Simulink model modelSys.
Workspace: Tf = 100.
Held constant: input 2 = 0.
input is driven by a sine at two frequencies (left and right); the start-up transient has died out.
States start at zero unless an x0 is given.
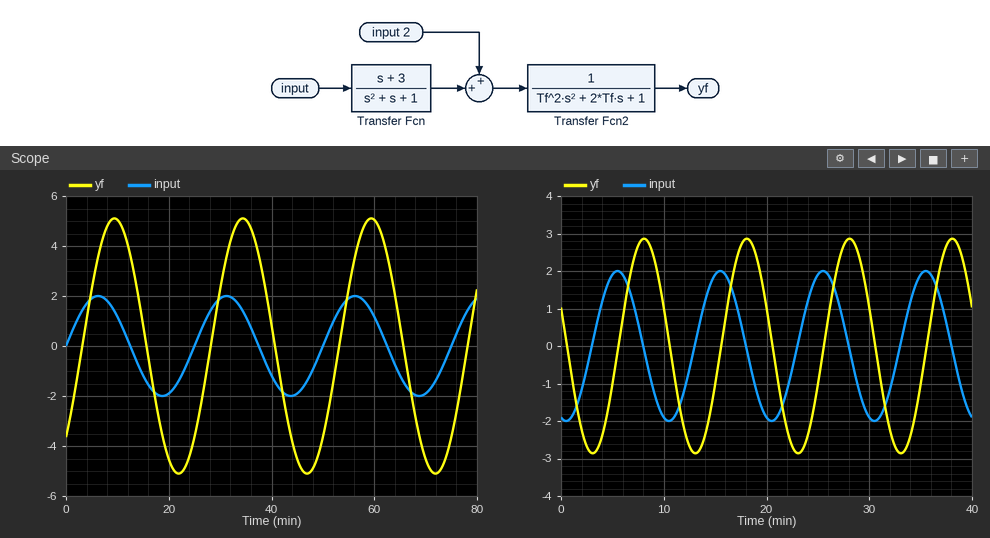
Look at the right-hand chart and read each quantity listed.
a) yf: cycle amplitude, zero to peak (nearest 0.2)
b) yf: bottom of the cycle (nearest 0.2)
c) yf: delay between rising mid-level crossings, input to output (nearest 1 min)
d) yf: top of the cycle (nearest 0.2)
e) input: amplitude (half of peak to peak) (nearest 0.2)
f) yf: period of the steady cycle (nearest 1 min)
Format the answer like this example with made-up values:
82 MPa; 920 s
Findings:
2.8; -2.8; 3 min; 2.8; 2.0; 10 min
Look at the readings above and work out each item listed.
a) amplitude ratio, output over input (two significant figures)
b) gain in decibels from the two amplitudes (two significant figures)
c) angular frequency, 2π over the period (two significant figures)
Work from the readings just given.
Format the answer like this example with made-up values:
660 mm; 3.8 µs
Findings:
1.4; 2.9 dB; 0.63 rad/min
